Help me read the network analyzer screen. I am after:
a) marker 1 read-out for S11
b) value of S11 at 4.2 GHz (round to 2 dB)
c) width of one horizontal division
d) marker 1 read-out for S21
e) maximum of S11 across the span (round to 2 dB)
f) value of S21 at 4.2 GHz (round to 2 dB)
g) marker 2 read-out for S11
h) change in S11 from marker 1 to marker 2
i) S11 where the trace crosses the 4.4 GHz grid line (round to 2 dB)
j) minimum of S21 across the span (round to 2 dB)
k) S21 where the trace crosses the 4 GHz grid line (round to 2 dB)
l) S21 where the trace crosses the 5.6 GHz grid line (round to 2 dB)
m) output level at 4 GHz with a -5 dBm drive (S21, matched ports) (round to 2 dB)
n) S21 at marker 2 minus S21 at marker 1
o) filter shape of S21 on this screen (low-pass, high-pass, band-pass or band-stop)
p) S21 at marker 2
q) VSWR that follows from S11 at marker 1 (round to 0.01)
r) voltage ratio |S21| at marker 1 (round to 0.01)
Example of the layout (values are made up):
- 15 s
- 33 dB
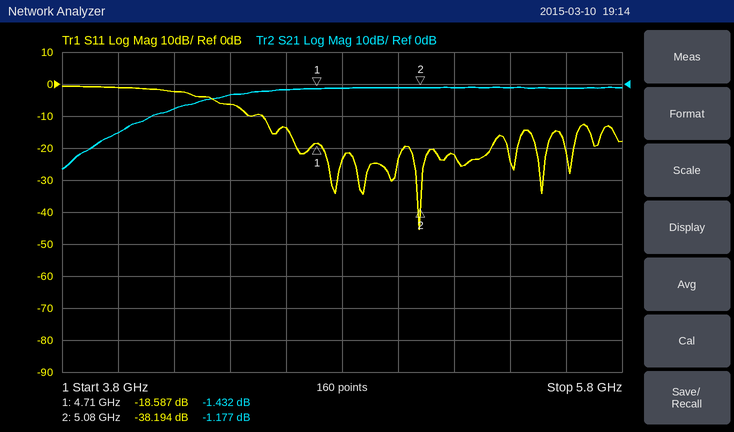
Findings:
- -18.587 dB
- -2 dB
- 200 MHz
- -1.432 dB
- 0 dB
- -8 dB
- -38.194 dB
- -19.607 dB
- -6 dB
- -26 dB
- -16 dB
- -2 dB
- -20 dBm
- 0.255 dB
- high-pass
- -1.177 dB
- 1.27
- 0.85
